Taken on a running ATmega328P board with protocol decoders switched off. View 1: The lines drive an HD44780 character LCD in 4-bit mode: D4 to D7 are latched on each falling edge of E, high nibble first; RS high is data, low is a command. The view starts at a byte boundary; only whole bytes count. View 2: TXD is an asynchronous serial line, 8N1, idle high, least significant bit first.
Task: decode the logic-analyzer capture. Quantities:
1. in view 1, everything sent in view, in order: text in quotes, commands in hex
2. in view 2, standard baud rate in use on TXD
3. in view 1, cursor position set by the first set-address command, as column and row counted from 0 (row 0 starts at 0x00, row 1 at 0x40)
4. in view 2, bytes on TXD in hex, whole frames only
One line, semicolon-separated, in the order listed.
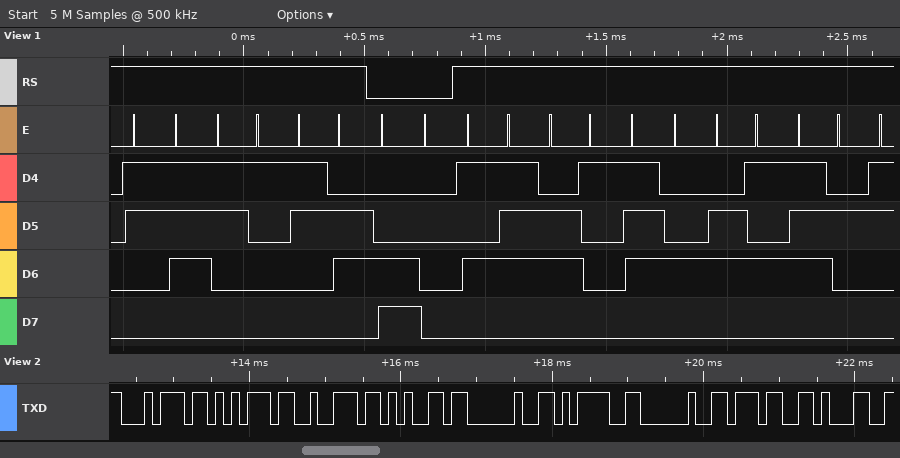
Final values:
"716" 0xC0 "Water"; 9600 baud; column 0, row 1; 74 75 72 65 20 3D 20 37 31
